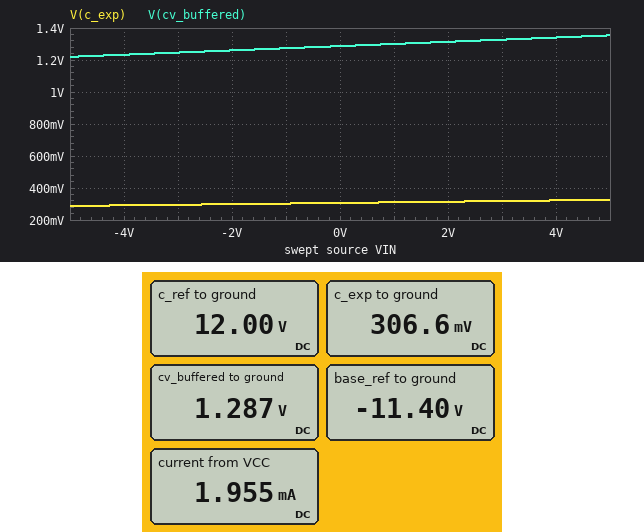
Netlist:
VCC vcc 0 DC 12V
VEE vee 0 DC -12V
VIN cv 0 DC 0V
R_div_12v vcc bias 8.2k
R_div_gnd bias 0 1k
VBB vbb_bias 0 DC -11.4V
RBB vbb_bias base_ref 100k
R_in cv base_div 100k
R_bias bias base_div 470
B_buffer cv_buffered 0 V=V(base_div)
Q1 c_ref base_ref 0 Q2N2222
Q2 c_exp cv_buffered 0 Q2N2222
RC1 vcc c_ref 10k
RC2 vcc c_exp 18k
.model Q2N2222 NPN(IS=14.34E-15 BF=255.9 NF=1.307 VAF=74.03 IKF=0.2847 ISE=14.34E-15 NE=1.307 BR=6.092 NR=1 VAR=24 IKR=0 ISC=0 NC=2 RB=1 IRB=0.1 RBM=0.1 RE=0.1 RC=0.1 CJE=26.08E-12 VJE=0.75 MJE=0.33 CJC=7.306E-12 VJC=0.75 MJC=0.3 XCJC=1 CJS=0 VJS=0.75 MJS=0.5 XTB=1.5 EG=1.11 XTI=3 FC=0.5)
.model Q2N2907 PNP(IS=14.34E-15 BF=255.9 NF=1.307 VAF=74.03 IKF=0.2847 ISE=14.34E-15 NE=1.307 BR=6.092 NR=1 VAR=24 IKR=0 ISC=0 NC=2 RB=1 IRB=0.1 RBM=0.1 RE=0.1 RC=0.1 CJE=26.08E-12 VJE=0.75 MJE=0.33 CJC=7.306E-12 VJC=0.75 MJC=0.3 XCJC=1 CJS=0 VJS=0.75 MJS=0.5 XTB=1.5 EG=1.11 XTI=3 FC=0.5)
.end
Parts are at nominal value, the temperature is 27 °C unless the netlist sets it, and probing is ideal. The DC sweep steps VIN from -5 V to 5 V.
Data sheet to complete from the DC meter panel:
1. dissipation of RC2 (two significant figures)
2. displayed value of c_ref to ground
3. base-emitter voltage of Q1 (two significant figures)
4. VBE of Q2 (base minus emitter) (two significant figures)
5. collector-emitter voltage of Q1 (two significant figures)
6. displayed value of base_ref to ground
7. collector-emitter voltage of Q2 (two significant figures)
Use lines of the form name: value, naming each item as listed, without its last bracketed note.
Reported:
dissipation of RC2: 7.6 mW
displayed value of c_ref to ground: 12.00 V
base-emitter voltage of Q1: -11 V
VBE of Q2 (base minus emitter): 1.3 V
collector-emitter voltage of Q1: 12 V
displayed value of base_ref to ground: -11.40 V
collector-emitter voltage of Q2: 310 mV
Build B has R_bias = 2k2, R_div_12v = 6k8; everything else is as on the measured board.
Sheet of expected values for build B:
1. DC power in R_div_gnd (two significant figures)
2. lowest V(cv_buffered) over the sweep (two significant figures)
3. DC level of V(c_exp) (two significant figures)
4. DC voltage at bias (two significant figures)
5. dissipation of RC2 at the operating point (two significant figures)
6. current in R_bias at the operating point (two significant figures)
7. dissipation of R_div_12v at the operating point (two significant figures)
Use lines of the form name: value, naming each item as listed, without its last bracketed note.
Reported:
DC power in R_div_gnd: 2.3 mW
lowest V(cv_buffered) over the sweep: 1.3 V
DC level of V(c_exp): 370 mV
DC voltage at bias: 1.5 V
dissipation of RC2 at the operating point: 7.5 mW
current in R_bias at the operating point: 15 µA
dissipation of R_div_12v at the operating point: 16 mW
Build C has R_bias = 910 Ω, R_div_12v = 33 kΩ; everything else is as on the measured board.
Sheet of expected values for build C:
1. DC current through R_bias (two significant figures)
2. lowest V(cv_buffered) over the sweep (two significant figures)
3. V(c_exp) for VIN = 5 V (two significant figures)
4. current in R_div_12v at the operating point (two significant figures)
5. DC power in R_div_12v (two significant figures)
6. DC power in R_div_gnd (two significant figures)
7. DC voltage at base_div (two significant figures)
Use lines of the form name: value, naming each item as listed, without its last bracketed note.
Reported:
DC current through R_bias: 3.5 µA
lowest V(cv_buffered) over the sweep: 250 mV
V(c_exp) for VIN = 5 V: 12 V
current in R_div_12v at the operating point: 350 µA
DC power in R_div_12v: 4.1 mW
DC power in R_div_gnd: 120 µW
DC voltage at base_div: 350 mV
